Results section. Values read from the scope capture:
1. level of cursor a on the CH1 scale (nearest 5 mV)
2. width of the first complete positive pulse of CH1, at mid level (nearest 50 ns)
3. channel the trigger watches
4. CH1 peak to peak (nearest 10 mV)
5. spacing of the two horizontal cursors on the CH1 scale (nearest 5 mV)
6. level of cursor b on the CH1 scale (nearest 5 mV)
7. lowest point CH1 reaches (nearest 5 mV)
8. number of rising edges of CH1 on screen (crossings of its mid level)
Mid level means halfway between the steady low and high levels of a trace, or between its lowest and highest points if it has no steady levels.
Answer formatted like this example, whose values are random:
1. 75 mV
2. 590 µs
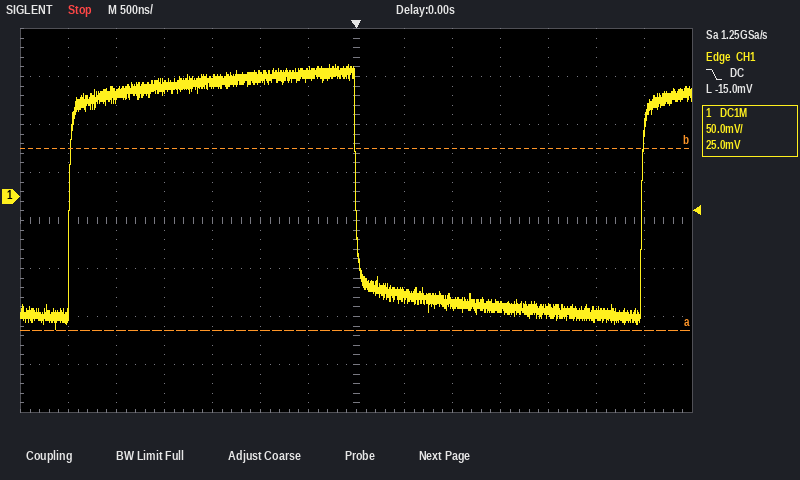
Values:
1. -140 mV
2. 3.00 µs
3. CH1
4. 280 mV
5. 190 mV
6. 50 mV
7. -140 mV
8. 2
